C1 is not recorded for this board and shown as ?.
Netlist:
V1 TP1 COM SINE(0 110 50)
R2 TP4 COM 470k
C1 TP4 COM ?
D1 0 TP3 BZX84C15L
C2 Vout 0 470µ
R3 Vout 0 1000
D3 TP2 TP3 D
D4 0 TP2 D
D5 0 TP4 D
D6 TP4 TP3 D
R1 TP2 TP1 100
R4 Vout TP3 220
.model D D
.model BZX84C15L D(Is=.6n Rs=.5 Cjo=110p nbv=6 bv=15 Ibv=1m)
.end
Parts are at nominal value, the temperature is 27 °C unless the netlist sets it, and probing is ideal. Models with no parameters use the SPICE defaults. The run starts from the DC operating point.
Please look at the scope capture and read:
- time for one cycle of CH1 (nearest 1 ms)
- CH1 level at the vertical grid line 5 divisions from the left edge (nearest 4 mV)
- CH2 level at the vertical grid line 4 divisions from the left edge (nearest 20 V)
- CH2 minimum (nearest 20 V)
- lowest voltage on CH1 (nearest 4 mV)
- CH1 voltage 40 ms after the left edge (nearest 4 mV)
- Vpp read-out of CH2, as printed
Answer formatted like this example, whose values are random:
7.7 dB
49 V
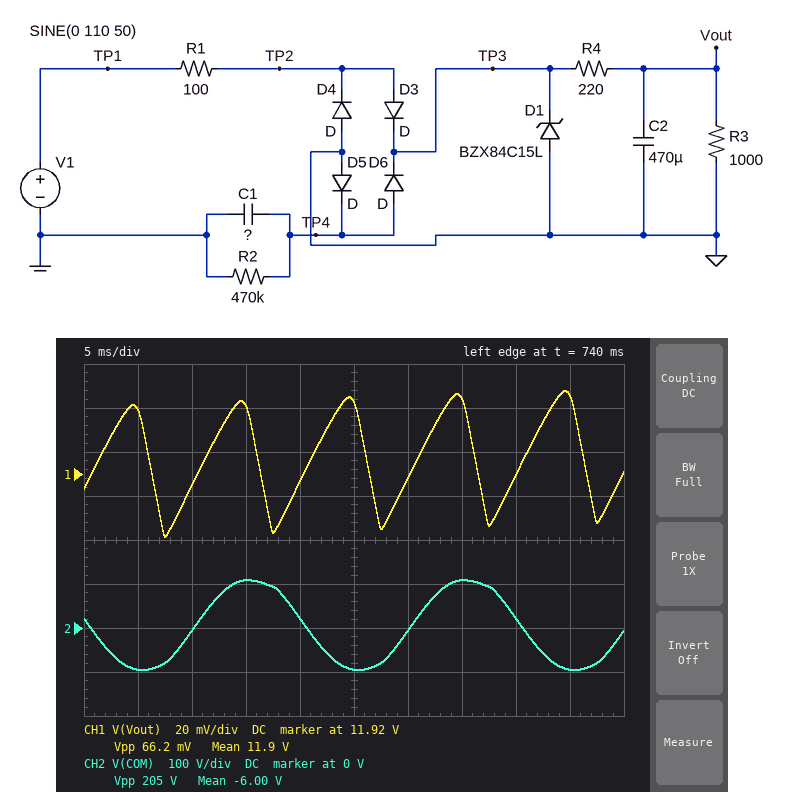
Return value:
10 ms
11.952 V
20 V
-100 V
11.892 V
11.920 V
205 V
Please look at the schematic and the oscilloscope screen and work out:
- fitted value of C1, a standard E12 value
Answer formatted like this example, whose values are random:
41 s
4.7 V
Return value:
1.5 µF
